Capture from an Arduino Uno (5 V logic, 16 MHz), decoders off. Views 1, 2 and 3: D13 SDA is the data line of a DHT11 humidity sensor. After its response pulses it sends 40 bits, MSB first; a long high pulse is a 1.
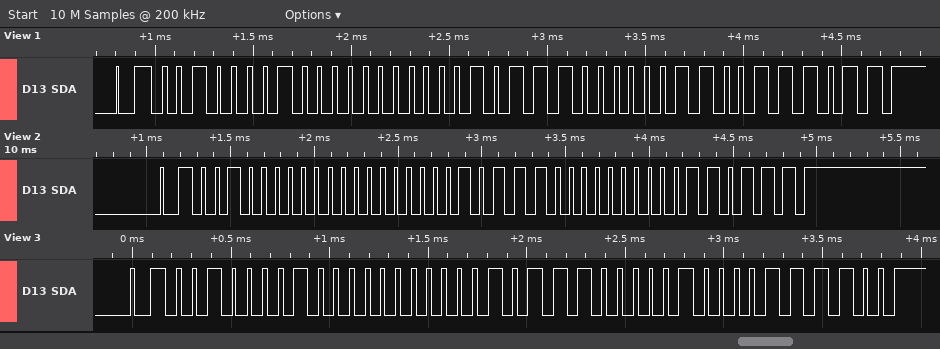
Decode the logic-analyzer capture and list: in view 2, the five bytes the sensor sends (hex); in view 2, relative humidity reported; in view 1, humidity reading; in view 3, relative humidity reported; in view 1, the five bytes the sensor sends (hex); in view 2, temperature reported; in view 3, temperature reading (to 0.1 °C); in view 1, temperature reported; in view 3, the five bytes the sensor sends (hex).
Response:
20 00 17 00 37
32 %
33 %
33 %
21 00 17 03 3B
23.0 °C
23.4 °C
23.3 °C
21 00 17 04 3C
